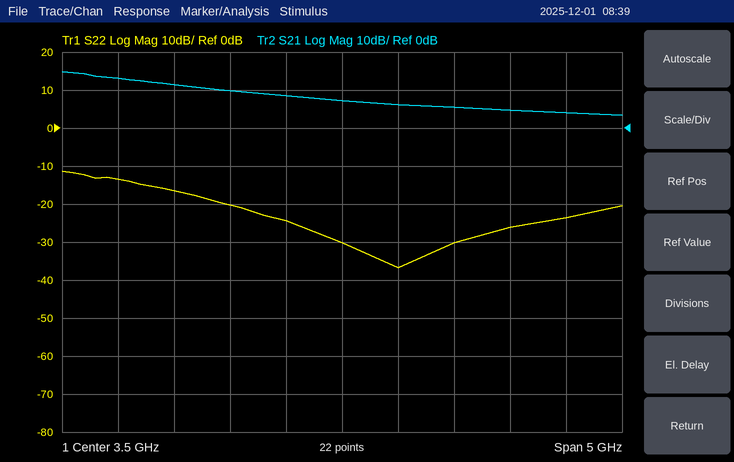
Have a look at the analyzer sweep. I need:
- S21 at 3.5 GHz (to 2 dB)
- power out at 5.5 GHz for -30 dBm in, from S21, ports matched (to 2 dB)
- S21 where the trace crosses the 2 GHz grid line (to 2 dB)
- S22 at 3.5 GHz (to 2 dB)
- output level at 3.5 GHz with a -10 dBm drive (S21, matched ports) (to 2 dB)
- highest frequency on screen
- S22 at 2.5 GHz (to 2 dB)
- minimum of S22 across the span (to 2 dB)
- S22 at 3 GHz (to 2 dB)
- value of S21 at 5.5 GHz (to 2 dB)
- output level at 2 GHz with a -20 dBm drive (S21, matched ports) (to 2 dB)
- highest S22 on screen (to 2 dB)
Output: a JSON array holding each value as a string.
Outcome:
["8 dB", "-26 dBm", "12 dB", "-30 dB", "-2 dBm", "6 GHz", "-20 dB", "-36 dB", "-24 dB", "4 dB", "-8 dBm", "-12 dB"]
